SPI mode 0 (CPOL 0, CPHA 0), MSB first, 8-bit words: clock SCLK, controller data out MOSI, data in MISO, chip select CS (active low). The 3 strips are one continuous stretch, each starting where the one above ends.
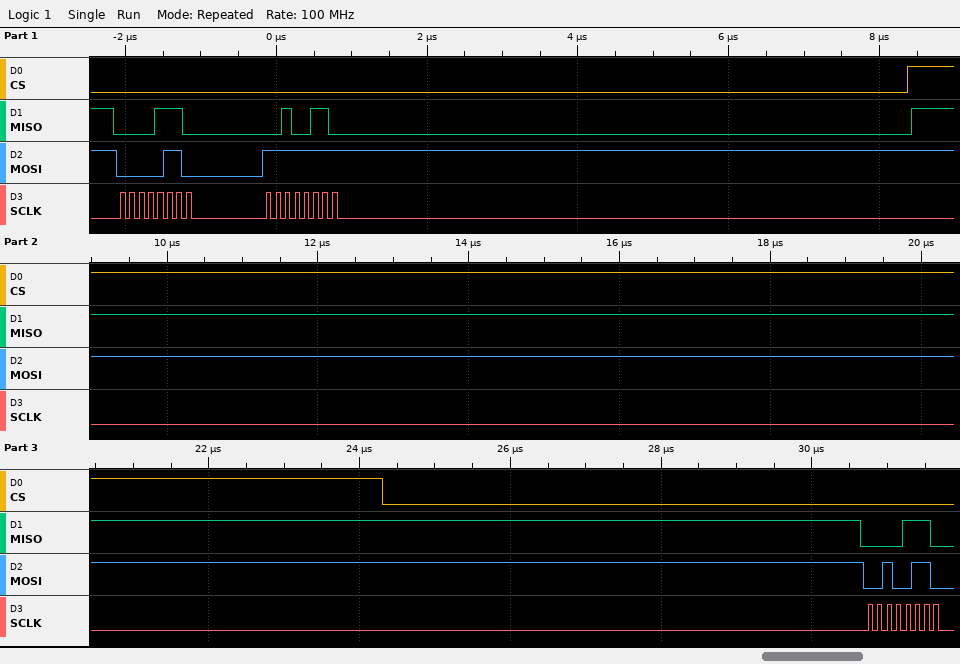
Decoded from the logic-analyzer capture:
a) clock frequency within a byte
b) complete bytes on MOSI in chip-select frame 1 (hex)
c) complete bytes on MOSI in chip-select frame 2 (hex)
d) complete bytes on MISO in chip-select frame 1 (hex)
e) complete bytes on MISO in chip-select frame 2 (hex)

8 MHz
06 FF
26
0E 26
0E
